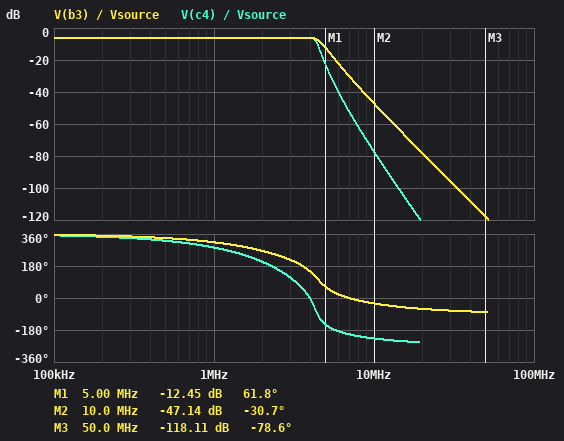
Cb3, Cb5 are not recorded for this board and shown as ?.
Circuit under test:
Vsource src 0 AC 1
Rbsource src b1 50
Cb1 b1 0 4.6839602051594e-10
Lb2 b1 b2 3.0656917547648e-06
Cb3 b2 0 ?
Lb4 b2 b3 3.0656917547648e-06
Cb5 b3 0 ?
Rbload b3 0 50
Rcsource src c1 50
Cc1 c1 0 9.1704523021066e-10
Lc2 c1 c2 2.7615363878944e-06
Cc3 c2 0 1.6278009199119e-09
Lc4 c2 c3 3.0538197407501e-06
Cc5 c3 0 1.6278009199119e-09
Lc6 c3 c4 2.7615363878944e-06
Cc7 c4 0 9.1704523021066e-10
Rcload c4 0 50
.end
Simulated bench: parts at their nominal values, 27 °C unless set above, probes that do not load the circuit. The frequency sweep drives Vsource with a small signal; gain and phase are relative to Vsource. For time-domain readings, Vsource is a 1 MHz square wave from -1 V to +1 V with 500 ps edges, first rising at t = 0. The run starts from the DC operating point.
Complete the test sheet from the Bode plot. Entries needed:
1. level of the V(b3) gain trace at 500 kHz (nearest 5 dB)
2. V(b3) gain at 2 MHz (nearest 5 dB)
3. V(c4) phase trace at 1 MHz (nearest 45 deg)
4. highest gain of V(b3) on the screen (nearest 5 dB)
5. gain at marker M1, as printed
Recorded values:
-5 dB
-5 dB
270 deg
-5 dB
-12.45 dB
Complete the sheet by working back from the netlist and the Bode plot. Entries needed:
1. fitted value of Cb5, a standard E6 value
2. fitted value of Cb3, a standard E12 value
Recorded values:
1 nF
1.2 nF
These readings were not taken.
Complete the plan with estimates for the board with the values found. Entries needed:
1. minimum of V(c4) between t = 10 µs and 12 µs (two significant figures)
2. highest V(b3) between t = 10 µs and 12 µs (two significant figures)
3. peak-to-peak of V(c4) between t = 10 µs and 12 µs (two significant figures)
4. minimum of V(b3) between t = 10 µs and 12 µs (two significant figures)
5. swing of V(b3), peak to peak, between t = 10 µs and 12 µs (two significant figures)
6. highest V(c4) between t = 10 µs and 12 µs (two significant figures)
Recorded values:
-650 mV
630 mV
1.3 V
-630 mV
1.3 V
650 mV
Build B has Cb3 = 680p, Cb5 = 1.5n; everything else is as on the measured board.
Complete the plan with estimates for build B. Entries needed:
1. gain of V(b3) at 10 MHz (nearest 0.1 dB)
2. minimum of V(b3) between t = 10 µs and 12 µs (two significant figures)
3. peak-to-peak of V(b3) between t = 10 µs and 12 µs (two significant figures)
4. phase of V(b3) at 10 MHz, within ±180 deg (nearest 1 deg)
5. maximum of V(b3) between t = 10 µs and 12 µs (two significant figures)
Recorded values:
-44.5 dB
-570 mV
1.1 V
-37 deg
570 mV
